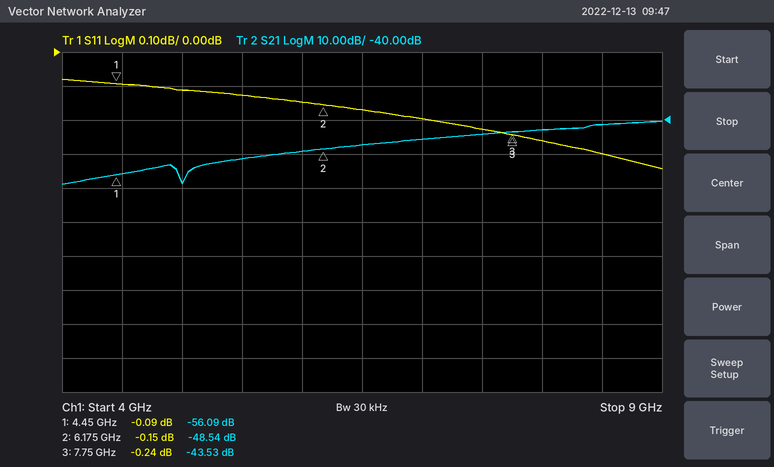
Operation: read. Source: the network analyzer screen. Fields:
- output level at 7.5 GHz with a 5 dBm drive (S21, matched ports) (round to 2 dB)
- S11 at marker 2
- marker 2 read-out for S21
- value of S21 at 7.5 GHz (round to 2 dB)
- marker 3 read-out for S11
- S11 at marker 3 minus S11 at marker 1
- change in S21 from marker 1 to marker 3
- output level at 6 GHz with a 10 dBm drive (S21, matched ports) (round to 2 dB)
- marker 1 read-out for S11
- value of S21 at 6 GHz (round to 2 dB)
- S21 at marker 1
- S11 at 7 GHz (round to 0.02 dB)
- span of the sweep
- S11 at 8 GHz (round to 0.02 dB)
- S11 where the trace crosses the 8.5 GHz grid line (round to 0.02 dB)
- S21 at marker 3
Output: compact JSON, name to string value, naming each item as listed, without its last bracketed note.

{"output level at 7.5 GHz with a 5 dBm drive (S21, matched ports)": "-40 dBm", "S11 at marker 2": "-0.15 dB", "marker 2 read-out for S21": "-48.54 dB", "value of S21 at 7.5 GHz": "-44 dB", "marker 3 read-out for S11": "-0.24 dB", "S11 at marker 3 minus S11 at marker 1": "-0.15 dB", "change in S21 from marker 1 to marker 3": "12.56 dB", "output level at 6 GHz with a 10 dBm drive (S21, matched ports)": "-40 dBm", "marker 1 read-out for S11": "-0.09 dB", "value of S21 at 6 GHz": "-50 dB", "S21 at marker 1": "-56.09 dB", "S11 at 7 GHz": "-0.20 dB", "span of the sweep": "5 GHz", "S11 at 8 GHz": "-0.26 dB", "S11 where the trace crosses the 8.5 GHz grid line": "-0.30 dB", "S21 at marker 3": "-43.53 dB"}
